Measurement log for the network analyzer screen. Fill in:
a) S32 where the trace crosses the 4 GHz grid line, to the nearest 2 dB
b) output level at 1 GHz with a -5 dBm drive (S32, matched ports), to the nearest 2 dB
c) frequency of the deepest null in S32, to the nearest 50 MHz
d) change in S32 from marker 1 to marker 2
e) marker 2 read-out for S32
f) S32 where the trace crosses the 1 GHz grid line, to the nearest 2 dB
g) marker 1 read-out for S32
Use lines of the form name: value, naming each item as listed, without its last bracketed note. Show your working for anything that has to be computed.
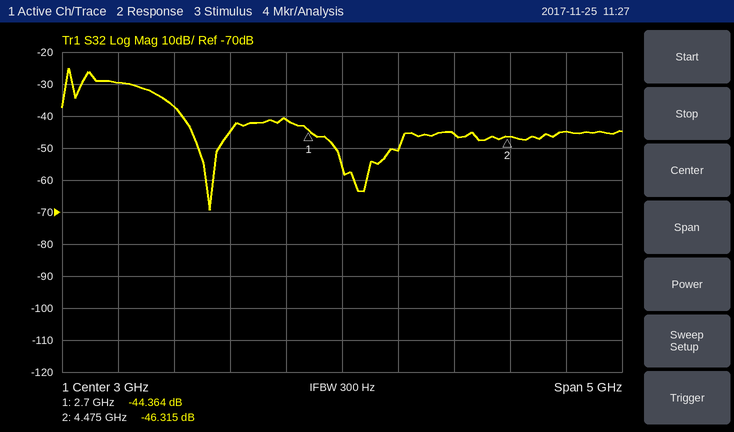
S32 where the trace crosses the 4 GHz grid line, to the nearest 2 dB: -46 dB
output level at 1 GHz with a -5 dBm drive (S32, matched ports), to the nearest 2 dB: -5 dBm + (-30 dB) = -34 dBm
frequency of the deepest null in S32, to the nearest 50 MHz: 1.80 GHz
change in S32 from marker 1 to marker 2: -46.315 − (-44.364) = -1.951 dB
marker 2 read-out for S32: -46.315 dB
S32 where the trace crosses the 1 GHz grid line, to the nearest 2 dB: -30 dB
marker 1 read-out for S32: -44.364 dB
